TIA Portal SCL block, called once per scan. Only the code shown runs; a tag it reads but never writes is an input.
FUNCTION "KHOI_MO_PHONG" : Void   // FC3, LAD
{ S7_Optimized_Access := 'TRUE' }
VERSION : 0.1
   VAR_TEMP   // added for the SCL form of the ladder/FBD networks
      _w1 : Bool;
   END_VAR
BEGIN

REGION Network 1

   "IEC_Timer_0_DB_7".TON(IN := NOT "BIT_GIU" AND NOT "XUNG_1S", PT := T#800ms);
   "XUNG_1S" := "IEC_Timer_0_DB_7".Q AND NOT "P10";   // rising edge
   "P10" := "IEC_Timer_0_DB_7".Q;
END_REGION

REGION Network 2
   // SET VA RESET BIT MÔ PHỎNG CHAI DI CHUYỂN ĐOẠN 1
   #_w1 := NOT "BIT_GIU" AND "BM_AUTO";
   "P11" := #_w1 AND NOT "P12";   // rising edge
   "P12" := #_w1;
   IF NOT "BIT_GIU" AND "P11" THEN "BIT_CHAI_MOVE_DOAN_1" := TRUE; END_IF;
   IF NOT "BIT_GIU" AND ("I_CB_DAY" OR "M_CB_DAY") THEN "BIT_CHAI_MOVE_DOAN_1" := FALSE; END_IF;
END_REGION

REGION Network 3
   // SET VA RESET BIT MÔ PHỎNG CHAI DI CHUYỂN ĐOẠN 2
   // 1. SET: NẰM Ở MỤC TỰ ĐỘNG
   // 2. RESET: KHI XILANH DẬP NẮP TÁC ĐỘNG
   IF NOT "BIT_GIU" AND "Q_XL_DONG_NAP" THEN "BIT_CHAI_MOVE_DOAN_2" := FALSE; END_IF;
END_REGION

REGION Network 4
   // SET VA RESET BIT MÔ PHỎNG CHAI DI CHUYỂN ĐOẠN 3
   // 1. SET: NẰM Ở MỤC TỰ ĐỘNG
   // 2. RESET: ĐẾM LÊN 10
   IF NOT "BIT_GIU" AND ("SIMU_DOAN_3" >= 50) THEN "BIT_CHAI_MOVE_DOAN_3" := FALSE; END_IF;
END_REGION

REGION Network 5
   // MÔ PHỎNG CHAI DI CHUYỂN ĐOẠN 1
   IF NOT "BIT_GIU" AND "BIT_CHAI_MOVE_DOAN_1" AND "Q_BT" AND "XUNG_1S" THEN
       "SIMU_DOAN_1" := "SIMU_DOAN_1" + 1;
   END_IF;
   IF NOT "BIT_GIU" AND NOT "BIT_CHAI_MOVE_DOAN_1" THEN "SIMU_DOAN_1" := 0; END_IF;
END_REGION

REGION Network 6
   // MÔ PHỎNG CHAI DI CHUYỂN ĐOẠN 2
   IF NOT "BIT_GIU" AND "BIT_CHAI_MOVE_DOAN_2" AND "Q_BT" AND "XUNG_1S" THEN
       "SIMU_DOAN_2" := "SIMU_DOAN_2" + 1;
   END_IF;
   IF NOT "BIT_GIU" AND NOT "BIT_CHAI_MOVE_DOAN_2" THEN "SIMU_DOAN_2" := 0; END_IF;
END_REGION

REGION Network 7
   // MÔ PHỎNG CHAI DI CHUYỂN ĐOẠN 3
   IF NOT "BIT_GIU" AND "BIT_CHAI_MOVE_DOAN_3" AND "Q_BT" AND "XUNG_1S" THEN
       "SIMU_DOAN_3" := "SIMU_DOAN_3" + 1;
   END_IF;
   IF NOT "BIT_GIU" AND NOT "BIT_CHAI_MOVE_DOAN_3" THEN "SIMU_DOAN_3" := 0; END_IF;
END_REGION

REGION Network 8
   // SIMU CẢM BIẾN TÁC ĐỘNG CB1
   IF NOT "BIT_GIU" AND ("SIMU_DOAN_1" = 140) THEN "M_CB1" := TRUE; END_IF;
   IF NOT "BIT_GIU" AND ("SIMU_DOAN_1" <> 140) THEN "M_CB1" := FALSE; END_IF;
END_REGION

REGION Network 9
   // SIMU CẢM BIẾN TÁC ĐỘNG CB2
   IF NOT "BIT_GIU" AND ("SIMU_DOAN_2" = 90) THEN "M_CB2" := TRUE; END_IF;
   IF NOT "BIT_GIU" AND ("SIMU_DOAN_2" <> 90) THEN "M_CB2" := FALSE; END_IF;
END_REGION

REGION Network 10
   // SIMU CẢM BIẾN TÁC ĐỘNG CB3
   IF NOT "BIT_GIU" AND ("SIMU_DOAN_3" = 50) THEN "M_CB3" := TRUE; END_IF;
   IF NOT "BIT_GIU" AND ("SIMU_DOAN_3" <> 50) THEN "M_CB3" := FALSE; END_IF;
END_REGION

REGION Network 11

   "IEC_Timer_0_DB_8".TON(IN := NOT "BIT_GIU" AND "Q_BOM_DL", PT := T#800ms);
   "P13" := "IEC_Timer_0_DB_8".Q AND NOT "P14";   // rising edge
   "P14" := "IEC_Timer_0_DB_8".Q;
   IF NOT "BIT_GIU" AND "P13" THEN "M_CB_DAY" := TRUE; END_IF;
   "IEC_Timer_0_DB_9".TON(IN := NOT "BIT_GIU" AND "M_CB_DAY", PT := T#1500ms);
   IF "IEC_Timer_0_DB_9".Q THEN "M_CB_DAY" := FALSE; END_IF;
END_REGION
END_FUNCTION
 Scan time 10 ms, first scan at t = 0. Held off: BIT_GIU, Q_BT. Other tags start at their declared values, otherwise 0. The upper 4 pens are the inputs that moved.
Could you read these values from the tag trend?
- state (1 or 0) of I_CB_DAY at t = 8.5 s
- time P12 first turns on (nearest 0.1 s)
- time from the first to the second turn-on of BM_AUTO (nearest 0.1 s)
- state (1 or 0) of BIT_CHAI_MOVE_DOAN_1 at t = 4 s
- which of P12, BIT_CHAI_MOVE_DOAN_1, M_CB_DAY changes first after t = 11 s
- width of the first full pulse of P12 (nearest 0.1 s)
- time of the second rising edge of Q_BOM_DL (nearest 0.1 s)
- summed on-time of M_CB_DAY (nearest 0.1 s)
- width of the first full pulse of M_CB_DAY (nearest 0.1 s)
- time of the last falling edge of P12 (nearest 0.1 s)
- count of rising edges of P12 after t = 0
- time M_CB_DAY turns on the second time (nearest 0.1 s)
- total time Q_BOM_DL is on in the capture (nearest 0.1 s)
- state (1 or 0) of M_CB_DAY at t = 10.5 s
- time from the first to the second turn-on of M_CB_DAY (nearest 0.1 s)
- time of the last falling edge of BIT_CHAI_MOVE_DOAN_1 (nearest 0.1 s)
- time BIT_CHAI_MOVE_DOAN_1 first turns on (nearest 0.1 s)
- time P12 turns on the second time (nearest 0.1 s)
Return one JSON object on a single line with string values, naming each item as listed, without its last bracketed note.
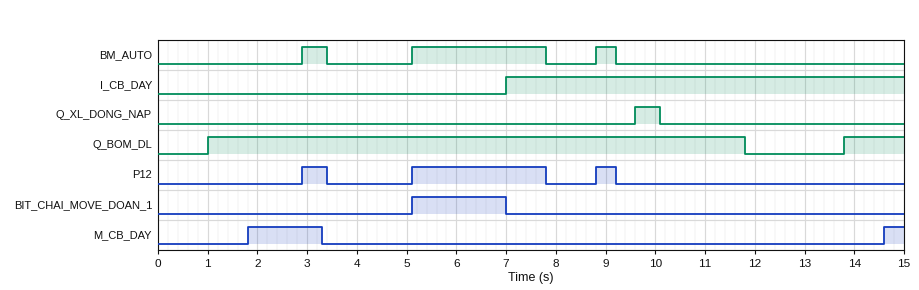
{"state (1 or 0) of I_CB_DAY at t = 8.5 s": "1", "time P12 first turns on": "2.9 s", "time from the first to the second turn-on of BM_AUTO": "2.2 s", "state (1 or 0) of BIT_CHAI_MOVE_DOAN_1 at t = 4 s": "0", "which of P12, BIT_CHAI_MOVE_DOAN_1, M_CB_DAY changes first after t = 11 s": "M_CB_DAY", "width of the first full pulse of P12": "0.5 s", "time of the second rising edge of Q_BOM_DL": "13.8 s", "summed on-time of M_CB_DAY": "1.9 s", "width of the first full pulse of M_CB_DAY": "1.5 s", "time of the last falling edge of P12": "9.2 s", "count of rising edges of P12 after t = 0": "3", "time M_CB_DAY turns on the second time": "14.6 s", "total time Q_BOM_DL is on in the capture": "12.0 s", "state (1 or 0) of M_CB_DAY at t = 10.5 s": "0", "time from the first to the second turn-on of M_CB_DAY": "12.8 s", "time of the last falling edge of BIT_CHAI_MOVE_DOAN_1": "7.0 s", "time BIT_CHAI_MOVE_DOAN_1 first turns on": "5.1 s", "time P12 turns on the second time": "5.1 s"}
